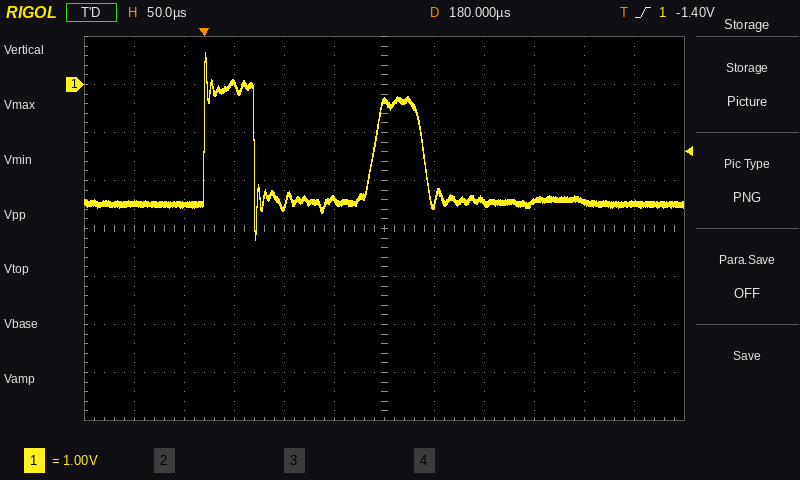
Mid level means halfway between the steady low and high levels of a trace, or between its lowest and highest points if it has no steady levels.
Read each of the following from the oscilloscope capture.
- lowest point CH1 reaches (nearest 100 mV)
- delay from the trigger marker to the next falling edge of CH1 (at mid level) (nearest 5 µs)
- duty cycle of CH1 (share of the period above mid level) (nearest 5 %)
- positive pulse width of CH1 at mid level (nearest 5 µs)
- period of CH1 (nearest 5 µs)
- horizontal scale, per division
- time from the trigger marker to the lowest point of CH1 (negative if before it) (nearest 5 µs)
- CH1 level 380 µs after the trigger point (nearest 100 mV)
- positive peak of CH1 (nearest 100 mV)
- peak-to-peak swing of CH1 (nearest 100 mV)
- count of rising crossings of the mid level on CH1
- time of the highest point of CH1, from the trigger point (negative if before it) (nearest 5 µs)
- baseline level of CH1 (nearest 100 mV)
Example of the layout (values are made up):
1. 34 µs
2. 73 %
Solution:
1. -3.2 V
2. 50 µs
3. 30 %
4. 50 µs
5. 170 µs
6. 50 µs
7. +50 µs
8. -2.4 V
9. 700 mV
10. 3.9 V
11. 2
12. 0 µs
13. -2.5 V
